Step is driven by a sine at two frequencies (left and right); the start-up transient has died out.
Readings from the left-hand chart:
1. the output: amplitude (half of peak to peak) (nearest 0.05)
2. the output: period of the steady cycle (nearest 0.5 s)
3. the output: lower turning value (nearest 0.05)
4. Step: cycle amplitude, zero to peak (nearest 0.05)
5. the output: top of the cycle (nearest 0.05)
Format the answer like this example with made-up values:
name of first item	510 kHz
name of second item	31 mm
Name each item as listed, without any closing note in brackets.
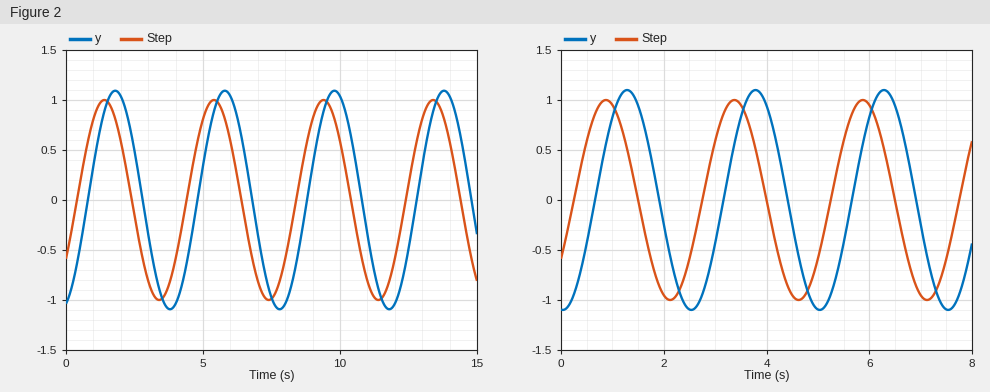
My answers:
the output: amplitude (half of peak to peak)	1.10
the output: period of the steady cycle	4.0 s
the output: lower turning value	-1.10
Step: cycle amplitude, zero to peak	1.00
the output: top of the cycle	1.10
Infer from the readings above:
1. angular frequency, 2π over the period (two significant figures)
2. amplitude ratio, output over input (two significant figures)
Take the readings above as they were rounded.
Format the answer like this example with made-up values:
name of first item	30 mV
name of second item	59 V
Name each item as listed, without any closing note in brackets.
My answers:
angular frequency, 2π over the period	1.6 rad/s
amplitude ratio, output over input	1.1
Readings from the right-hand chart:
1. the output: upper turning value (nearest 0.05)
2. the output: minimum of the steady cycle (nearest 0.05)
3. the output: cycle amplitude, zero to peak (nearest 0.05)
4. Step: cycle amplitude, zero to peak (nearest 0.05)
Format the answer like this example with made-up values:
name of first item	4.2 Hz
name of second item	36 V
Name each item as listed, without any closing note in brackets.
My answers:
the output: upper turning value	1.10
the output: minimum of the steady cycle	-1.10
the output: cycle amplitude, zero to peak	1.10
Step: cycle amplitude, zero to peak	1.00
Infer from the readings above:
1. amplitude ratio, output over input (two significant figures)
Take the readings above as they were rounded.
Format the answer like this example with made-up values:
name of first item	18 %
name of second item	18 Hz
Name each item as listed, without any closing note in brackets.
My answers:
amplitude ratio, output over input	1.1
